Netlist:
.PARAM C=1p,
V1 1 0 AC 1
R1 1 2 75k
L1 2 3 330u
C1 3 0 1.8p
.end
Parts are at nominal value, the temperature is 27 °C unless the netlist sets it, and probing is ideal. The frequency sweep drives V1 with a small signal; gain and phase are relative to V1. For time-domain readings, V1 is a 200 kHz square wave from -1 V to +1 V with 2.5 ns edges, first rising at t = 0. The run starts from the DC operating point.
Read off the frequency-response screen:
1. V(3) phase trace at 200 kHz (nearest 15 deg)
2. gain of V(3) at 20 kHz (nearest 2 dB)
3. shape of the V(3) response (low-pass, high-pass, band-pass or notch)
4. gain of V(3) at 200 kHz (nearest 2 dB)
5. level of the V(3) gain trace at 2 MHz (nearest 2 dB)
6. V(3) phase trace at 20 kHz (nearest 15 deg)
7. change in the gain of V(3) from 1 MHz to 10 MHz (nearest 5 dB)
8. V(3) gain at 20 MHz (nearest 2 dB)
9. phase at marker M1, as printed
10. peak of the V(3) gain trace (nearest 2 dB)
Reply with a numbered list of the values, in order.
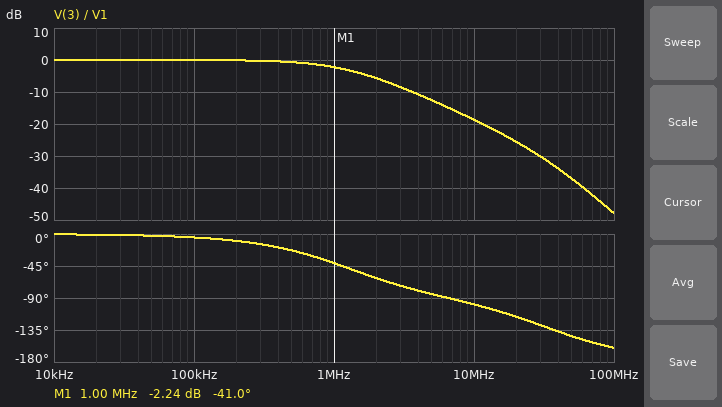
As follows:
1. -15 deg
2. 0 dB
3. low-pass
4. 0 dB
5. -6 dB
6. 0 deg
7. -15 dB
8. -26 dB
9. -41.0 deg
10. 0 dB
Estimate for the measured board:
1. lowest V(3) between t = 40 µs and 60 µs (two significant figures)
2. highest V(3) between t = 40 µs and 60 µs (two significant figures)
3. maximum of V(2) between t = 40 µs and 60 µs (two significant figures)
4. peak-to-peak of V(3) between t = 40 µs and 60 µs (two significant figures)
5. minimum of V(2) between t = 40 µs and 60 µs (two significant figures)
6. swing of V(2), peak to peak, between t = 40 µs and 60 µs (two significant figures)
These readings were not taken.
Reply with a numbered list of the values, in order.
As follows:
1. -1.0 V
2. 1.0 V
3. 1.0 V
4. 2.0 V
5. -1.0 V
6. 2.0 V
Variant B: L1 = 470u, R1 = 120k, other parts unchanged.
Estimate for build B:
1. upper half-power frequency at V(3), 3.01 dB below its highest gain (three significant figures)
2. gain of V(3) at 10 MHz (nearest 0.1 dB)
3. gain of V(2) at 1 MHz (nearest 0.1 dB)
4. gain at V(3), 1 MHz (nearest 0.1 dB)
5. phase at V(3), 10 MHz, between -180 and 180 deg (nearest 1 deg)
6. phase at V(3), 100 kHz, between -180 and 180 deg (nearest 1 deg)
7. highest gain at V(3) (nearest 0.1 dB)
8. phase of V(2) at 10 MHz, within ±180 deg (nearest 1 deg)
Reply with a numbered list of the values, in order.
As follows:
1. 750 kHz
2. -22.8 dB
3. -4.7 dB
4. -4.4 dB
5. -100 deg
6. -8 deg
7. 0 dB
8. 80 deg
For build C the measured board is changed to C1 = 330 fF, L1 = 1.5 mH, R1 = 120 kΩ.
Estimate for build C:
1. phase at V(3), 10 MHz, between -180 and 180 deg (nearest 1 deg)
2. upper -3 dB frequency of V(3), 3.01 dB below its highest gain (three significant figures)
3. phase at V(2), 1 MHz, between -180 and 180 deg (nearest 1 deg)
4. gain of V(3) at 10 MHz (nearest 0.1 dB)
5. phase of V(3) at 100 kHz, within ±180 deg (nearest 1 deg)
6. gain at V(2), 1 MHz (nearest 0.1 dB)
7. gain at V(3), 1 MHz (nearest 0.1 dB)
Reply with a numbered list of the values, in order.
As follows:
1. -111 deg
2. 5.42 MHz
3. -14 deg
4. -8.5 dB
5. -1 deg
6. -0.3 dB
7. -0.1 dB
